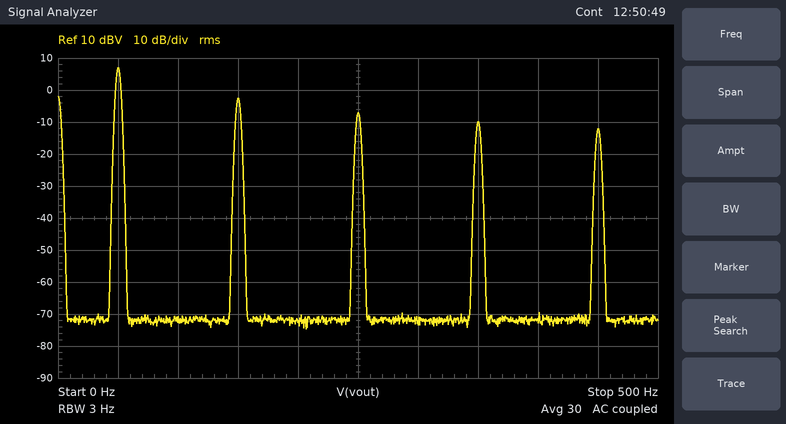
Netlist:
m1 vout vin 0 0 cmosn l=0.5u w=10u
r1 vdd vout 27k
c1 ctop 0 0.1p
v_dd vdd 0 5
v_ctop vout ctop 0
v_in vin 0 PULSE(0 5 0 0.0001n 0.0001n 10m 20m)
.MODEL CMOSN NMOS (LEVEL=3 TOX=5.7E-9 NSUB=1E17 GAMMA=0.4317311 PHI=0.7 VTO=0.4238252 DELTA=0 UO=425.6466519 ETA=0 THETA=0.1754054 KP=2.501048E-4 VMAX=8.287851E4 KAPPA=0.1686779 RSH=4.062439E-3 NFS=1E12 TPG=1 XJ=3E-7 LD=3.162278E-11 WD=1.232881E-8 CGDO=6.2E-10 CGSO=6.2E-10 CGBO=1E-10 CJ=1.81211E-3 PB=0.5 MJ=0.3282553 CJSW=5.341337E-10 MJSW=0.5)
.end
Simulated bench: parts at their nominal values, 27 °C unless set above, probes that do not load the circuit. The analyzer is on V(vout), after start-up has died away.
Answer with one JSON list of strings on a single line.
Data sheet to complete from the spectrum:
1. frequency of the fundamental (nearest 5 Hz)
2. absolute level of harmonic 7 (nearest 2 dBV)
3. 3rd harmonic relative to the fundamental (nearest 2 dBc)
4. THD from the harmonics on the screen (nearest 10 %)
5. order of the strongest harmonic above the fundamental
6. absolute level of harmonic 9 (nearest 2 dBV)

["50 Hz", "-10 dBV", "-10 dBc", "40 %", "3", "-12 dBV"]
